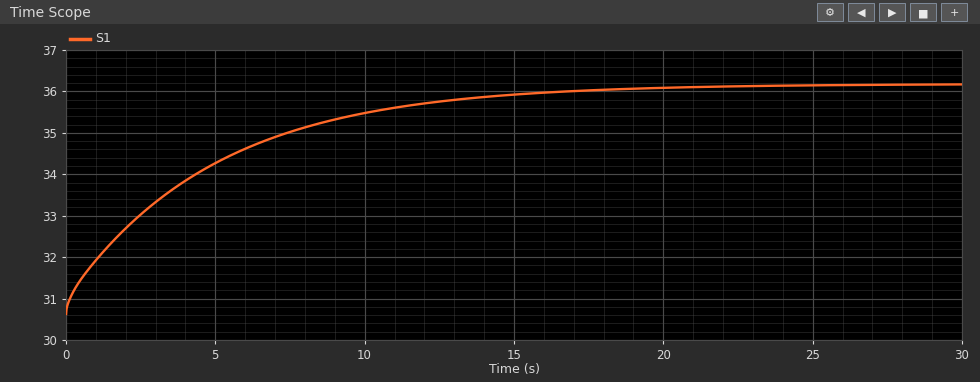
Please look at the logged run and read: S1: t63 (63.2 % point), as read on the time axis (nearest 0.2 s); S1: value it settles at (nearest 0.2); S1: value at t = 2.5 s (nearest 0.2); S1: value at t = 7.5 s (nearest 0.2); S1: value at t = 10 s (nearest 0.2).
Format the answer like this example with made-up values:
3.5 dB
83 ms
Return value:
4.6 s
36.2
33.0
35.0
35.4
